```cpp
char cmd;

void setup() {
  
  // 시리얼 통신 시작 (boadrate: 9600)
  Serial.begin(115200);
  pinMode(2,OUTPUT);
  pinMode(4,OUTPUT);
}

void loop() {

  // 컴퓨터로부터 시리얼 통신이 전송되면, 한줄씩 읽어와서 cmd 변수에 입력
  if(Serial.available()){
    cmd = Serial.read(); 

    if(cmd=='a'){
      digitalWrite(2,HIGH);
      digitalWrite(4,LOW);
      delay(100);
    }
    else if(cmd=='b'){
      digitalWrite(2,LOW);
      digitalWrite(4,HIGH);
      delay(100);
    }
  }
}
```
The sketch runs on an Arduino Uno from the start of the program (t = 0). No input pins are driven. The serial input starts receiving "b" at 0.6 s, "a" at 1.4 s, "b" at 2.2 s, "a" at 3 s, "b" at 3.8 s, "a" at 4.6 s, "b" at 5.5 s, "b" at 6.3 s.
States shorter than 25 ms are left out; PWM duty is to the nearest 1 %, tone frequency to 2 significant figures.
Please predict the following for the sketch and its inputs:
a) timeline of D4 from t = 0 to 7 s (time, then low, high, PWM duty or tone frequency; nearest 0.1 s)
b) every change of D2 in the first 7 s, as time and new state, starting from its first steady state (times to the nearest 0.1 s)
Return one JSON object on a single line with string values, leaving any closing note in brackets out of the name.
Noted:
{"timeline of D4 from t = 0 to 7 s": "0 s low; 0.6 s high; 1.4 s low; 2.2 s high; 3 s low; 3.8 s high; 4.6 s low; 5.5 s high", "every change of D2 in the first 7 s, as time and new state, starting from its first steady state": "0 s low; 1.4 s high; 2.2 s low; 3 s high; 3.8 s low; 4.6 s high; 5.5 s low"}
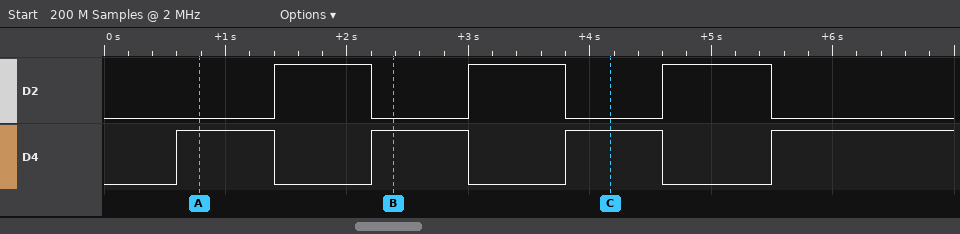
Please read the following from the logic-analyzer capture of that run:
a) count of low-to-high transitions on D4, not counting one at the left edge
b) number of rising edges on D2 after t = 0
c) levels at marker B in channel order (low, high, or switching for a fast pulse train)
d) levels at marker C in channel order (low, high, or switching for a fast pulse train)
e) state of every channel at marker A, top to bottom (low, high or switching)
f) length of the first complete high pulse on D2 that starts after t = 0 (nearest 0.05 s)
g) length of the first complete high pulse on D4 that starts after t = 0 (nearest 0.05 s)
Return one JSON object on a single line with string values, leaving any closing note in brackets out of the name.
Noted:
{"count of low-to-high transitions on D4, not counting one at the left edge": "4", "number of rising edges on D2 after t = 0": "3", "levels at marker B in channel order": "D2 low, D4 high", "levels at marker C in channel order": "D2 low, D4 high", "state of every channel at marker A, top to bottom": "D2 low, D4 high", "length of the first complete high pulse on D2 that starts after t = 0": "0.80 s", "length of the first complete high pulse on D4 that starts after t = 0": "0.80 s"}
